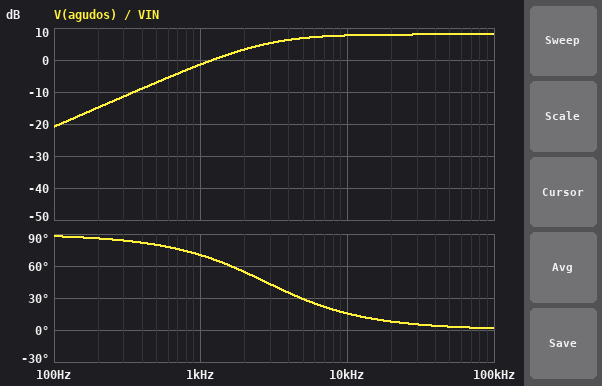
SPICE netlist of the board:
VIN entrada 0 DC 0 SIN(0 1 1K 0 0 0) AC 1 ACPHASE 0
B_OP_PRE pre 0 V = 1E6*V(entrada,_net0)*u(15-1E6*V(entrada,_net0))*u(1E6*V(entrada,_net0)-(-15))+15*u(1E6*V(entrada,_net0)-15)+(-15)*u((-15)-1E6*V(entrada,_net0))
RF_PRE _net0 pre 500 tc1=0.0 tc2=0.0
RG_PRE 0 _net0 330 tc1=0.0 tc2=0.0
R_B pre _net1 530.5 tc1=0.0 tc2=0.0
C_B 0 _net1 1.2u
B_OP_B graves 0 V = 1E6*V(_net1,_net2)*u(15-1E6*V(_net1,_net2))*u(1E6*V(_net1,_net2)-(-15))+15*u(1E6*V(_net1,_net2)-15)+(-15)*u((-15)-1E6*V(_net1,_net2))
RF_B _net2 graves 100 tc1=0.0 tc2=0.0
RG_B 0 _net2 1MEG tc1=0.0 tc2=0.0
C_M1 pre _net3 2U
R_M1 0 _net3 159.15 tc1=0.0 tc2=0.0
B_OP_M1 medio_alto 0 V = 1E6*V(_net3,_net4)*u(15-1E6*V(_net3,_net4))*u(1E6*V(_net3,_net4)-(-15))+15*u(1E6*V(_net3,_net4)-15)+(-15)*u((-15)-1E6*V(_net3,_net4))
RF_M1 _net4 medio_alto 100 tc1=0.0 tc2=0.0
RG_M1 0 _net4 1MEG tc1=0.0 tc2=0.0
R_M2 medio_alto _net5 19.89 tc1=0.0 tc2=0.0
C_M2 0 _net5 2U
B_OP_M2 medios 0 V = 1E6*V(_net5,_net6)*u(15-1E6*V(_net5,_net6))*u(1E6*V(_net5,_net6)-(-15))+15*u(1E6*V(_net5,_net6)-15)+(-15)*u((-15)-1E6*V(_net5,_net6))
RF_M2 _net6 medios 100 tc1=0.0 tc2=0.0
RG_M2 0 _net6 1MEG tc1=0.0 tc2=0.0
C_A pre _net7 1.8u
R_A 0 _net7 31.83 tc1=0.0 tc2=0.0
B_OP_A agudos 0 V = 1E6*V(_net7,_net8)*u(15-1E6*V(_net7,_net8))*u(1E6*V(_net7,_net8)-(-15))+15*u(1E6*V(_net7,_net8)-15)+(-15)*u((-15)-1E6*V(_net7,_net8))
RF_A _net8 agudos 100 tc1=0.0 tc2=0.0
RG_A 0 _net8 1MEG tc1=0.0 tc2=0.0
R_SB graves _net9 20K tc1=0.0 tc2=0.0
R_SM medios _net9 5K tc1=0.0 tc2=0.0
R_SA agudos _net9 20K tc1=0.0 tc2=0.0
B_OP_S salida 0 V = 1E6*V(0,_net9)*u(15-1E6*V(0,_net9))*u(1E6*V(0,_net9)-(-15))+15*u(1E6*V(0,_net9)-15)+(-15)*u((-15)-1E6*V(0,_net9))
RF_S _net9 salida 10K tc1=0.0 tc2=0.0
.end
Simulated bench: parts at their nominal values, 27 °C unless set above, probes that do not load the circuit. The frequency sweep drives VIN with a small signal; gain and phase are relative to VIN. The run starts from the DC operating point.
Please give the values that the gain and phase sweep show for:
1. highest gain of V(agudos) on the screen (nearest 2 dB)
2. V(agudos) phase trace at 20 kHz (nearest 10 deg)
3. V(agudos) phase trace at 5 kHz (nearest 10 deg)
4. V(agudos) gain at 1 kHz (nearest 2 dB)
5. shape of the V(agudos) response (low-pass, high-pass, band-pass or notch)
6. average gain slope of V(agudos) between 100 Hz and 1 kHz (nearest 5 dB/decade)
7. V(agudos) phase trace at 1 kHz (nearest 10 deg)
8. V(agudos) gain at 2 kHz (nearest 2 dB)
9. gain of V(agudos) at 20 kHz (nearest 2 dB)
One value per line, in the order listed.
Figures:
8 dB
10 deg
30 deg
-2 dB
high-pass
20 dB/decade
70 deg
4 dB
8 dB
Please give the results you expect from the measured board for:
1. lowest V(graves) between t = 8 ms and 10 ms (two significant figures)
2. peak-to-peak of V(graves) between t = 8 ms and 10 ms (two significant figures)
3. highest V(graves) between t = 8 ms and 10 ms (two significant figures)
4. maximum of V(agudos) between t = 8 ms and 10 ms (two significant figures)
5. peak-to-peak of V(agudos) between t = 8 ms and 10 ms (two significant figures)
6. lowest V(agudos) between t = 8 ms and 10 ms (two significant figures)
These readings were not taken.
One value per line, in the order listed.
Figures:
-610 mV
1.2 V
610 mV
850 mV
1.7 V
-850 mV
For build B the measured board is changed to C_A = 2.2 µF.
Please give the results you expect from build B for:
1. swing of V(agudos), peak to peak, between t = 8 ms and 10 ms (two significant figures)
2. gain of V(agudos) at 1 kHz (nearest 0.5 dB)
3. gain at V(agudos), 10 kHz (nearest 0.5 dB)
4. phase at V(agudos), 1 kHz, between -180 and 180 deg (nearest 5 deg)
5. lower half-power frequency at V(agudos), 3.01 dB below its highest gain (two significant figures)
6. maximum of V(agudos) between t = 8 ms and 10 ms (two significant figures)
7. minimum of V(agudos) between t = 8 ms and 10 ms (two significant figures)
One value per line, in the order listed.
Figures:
2.0 V
0 dB
8.0 dB
65 deg
2.3 kHz
1.0 V
-1.0 V
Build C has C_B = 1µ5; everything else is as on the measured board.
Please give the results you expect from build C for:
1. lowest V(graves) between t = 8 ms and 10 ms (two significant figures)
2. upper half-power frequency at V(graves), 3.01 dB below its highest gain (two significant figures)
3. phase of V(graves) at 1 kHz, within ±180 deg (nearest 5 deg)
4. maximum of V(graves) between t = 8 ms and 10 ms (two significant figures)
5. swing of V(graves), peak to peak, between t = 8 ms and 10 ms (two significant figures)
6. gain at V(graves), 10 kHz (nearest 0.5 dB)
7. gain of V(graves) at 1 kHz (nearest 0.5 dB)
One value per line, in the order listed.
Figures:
-490 mV
200 Hz
-80 deg
490 mV
990 mV
-26.0 dB
-6.0 dB
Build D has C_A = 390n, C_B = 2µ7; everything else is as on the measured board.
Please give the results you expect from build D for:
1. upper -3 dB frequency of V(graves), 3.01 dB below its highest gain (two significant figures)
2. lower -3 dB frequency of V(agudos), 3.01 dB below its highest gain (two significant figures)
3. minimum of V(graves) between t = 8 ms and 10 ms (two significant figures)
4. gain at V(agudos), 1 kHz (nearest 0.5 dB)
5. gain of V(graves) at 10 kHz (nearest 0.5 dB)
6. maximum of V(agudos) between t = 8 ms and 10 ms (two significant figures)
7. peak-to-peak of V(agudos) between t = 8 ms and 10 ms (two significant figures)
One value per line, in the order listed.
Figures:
110 Hz
13 kHz
-280 mV
-14.0 dB
-31.0 dB
200 mV
390 mV
